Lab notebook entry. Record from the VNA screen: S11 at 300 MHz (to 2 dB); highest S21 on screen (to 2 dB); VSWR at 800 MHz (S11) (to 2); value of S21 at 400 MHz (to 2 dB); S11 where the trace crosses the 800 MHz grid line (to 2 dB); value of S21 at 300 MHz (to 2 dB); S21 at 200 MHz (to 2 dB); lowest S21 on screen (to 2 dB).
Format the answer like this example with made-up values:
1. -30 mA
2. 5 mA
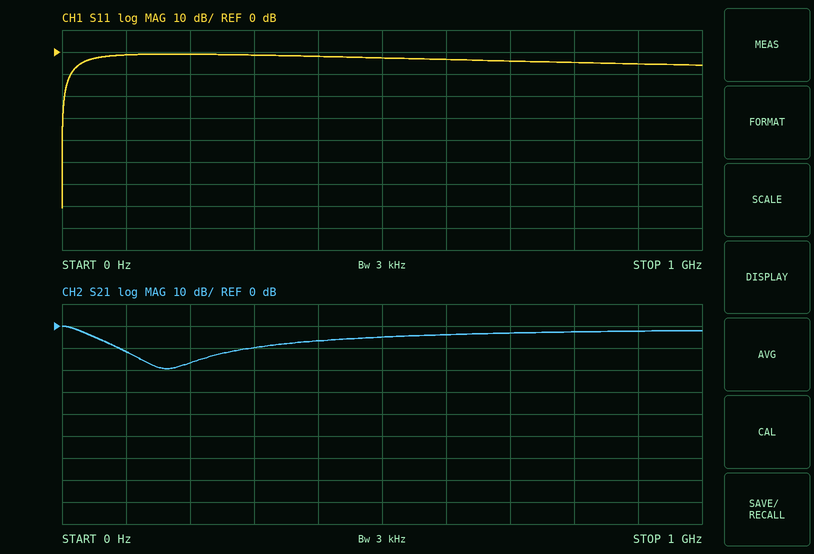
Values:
1. -2 dB
2. 0 dB
3. 4
4. -6 dB
5. -4 dB
6. -10 dB
7. -16 dB
8. -20 dB
